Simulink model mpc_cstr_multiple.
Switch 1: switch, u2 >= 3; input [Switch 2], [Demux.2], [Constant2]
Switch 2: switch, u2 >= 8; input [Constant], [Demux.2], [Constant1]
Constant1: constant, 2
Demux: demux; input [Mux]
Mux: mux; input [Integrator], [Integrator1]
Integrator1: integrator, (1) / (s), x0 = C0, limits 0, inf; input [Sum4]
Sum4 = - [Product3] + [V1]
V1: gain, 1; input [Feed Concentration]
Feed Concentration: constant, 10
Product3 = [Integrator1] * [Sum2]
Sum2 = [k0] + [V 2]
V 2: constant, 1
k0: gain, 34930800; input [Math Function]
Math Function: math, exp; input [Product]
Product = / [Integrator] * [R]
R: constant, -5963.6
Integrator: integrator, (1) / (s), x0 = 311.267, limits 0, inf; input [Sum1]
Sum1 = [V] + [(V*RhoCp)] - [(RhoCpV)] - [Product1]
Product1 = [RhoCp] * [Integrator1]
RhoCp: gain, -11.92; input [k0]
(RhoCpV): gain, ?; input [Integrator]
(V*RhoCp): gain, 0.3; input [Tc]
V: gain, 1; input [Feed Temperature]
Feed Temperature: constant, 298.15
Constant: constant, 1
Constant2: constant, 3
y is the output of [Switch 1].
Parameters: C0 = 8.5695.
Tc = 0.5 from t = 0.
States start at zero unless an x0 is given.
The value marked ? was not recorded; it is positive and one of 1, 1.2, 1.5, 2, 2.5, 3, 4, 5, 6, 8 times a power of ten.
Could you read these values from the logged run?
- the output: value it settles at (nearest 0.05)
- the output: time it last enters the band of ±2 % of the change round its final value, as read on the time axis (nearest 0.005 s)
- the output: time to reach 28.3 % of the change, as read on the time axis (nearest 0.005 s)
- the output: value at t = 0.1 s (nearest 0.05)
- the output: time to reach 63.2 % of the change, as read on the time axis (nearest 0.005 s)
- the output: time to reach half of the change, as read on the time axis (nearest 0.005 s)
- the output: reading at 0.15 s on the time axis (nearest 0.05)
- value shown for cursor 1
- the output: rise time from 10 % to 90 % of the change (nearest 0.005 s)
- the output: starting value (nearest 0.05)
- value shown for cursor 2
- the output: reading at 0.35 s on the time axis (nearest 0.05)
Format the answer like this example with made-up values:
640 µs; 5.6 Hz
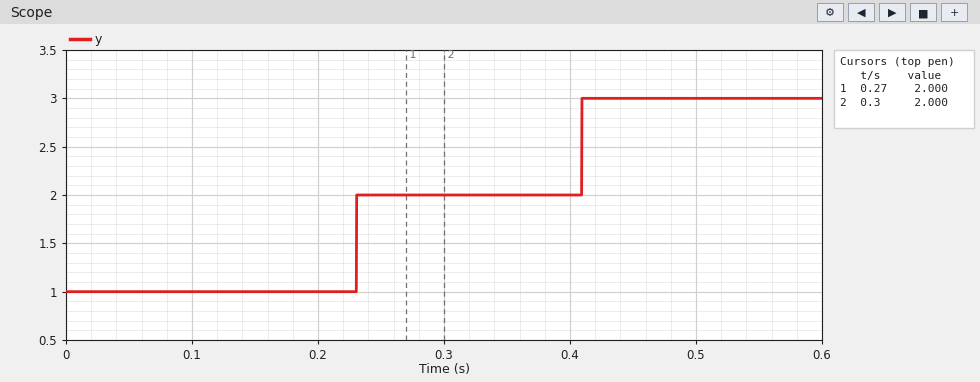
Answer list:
3.00; 0.410 s; 0.230 s; 1.00; 0.410 s; 0.230 s; 1.00; 2.000; 0.180 s; 1.00; 2.000; 2.00
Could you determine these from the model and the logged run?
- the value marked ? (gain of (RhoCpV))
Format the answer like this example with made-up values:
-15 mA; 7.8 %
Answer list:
0.6
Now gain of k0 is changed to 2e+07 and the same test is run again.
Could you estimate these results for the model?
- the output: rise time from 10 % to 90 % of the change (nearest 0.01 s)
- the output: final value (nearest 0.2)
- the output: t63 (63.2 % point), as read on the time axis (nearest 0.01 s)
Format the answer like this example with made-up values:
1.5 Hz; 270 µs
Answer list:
0.20 s; 3.0; 0.53 s
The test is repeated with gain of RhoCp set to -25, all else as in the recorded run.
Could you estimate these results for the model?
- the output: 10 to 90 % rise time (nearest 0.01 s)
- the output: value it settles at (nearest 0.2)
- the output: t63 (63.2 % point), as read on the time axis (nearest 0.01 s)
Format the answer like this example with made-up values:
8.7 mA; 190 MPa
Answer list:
0.08 s; 3.0; 0.27 s
